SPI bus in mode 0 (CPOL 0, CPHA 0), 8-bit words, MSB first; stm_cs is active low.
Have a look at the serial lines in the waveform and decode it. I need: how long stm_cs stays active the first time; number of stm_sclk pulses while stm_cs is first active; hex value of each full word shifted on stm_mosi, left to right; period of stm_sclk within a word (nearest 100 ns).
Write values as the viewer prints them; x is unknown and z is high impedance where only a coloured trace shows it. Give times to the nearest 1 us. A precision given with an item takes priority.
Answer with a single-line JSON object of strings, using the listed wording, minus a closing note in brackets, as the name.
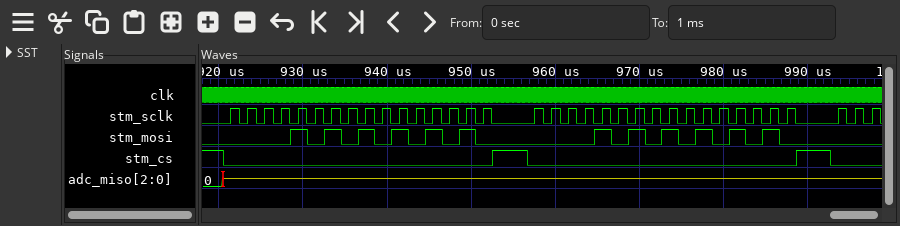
{"how long stm_cs stays active the first time": "32 us", "number of stm_sclk pulses while stm_cs is first active": "16", "hex value of each full word shifted on stm_mosi, left to right": "0A, AA, 0A, AA", "period of stm_sclk within a word": "2000 ns"}
